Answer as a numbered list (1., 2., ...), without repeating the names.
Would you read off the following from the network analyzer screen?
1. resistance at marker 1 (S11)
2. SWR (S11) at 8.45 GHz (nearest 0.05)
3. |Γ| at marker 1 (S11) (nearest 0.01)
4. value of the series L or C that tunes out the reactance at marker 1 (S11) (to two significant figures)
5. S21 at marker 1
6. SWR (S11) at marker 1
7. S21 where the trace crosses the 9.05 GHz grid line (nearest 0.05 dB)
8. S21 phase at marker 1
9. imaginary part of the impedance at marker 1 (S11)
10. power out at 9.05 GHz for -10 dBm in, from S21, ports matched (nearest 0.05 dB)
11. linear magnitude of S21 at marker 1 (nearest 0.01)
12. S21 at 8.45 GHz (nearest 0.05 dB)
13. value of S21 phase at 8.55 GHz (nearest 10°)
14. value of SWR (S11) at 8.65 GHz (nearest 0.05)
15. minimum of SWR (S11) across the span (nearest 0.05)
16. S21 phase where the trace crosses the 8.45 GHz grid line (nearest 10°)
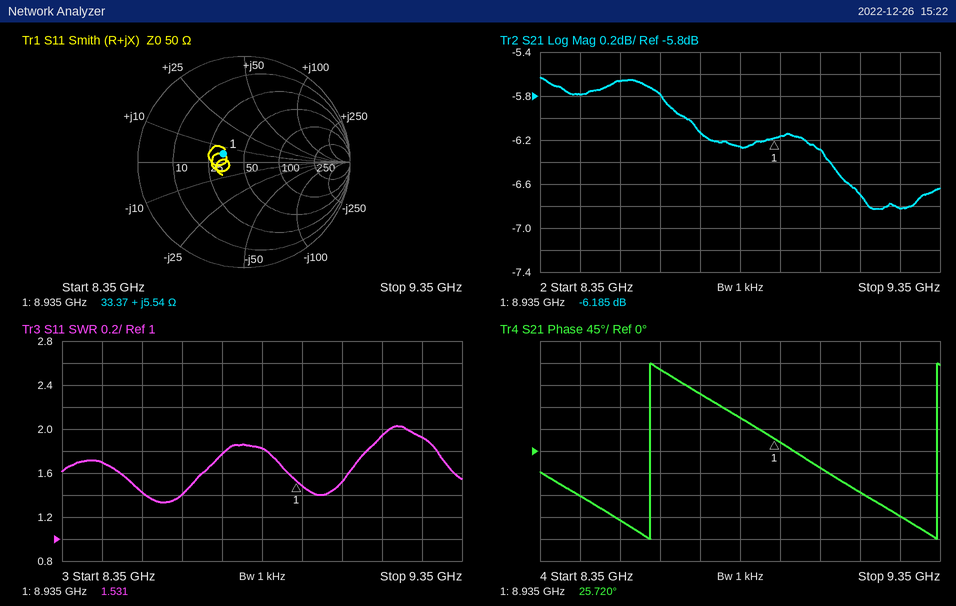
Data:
1. 33.37 Ω
2. 1.70
3. 0.21
4. 3.2 pF
5. -6.185 dB
6. 1.531
7. -6.30 dB
8. 25.720°
9. +5.54 Ω
10. -16.30 dBm
11. 0.49
12. -5.80 dB
13. -140°
14. 1.40
15. 1.35
16. -90°
